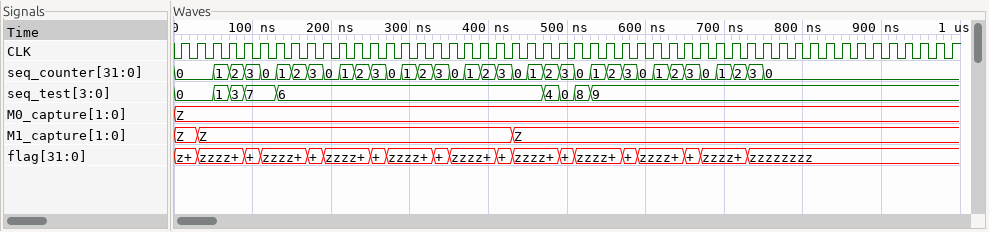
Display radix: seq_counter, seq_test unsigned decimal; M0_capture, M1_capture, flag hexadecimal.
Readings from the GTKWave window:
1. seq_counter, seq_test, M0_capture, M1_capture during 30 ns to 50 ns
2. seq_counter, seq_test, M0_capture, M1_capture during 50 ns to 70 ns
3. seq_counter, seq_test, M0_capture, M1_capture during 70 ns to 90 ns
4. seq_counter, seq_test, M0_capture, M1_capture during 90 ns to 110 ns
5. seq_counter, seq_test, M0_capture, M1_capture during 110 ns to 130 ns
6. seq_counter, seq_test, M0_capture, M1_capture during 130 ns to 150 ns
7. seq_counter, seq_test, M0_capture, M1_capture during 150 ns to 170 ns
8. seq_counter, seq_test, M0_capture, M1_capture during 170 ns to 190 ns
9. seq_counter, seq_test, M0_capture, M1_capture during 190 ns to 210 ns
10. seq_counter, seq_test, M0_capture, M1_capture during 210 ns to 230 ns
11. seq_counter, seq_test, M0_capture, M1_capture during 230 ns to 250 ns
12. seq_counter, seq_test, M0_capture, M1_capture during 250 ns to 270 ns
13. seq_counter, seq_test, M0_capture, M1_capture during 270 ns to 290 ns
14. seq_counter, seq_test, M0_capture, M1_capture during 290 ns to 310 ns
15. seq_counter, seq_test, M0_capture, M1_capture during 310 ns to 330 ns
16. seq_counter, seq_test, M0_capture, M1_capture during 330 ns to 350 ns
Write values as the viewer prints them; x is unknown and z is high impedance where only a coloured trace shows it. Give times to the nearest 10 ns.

seq_counter=0, seq_test=0, M0_capture=Z, M1_capture=Z
seq_counter=1, seq_test=1, M0_capture=Z, M1_capture=Z
seq_counter=2, seq_test=3, M0_capture=Z, M1_capture=Z
seq_counter=3, seq_test=7, M0_capture=Z, M1_capture=Z
seq_counter=0, seq_test=7, M0_capture=Z, M1_capture=Z
seq_counter=1, seq_test=6, M0_capture=Z, M1_capture=Z
seq_counter=2, seq_test=6, M0_capture=Z, M1_capture=Z
seq_counter=3, seq_test=6, M0_capture=Z, M1_capture=Z
seq_counter=0, seq_test=6, M0_capture=Z, M1_capture=Z
seq_counter=1, seq_test=6, M0_capture=Z, M1_capture=Z
seq_counter=2, seq_test=6, M0_capture=Z, M1_capture=Z
seq_counter=3, seq_test=6, M0_capture=Z, M1_capture=Z
seq_counter=0, seq_test=6, M0_capture=Z, M1_capture=Z
seq_counter=1, seq_test=6, M0_capture=Z, M1_capture=Z
seq_counter=2, seq_test=6, M0_capture=Z, M1_capture=Z
seq_counter=3, seq_test=6, M0_capture=Z, M1_capture=Z
